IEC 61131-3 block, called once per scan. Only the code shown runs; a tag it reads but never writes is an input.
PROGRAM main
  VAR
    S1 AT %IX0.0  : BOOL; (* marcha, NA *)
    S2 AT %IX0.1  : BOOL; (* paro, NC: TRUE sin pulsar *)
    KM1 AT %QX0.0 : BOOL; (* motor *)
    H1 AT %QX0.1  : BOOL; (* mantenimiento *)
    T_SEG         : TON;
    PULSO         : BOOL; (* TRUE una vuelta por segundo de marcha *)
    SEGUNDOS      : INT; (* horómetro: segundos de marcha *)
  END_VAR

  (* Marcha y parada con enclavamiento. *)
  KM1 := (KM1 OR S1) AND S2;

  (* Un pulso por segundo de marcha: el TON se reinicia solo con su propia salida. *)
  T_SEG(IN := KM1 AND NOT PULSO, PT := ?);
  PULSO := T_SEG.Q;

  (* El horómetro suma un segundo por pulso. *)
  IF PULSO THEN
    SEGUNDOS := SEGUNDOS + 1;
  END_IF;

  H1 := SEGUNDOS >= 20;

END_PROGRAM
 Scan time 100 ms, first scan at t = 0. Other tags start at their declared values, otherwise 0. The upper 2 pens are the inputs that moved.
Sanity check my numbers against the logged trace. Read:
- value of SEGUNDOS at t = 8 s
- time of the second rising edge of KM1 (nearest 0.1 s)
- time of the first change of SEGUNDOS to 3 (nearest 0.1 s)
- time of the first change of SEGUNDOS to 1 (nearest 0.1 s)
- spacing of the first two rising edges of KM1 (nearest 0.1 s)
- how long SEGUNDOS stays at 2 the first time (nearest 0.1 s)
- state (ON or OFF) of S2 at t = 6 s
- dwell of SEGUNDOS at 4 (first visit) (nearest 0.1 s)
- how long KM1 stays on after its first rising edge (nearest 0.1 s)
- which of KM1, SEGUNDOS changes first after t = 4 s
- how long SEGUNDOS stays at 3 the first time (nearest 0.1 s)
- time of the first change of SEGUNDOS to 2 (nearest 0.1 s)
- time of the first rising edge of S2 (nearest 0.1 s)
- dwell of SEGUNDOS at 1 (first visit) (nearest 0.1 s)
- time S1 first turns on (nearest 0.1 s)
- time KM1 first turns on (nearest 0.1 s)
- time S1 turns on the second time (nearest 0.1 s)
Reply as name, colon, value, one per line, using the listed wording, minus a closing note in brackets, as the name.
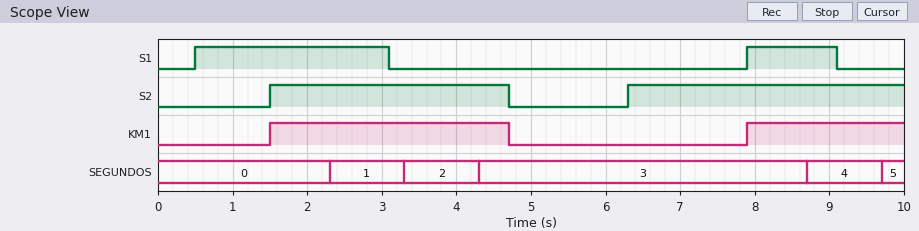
value of SEGUNDOS at t = 8 s: 3
time of the second rising edge of KM1: 7.9 s
time of the first change of SEGUNDOS to 3: 4.3 s
time of the first change of SEGUNDOS to 1: 2.3 s
spacing of the first two rising edges of KM1: 6.4 s
how long SEGUNDOS stays at 2 the first time: 1.0 s
state (ON or OFF) of S2 at t = 6 s: OFF
dwell of SEGUNDOS at 4 (first visit): 1.0 s
how long KM1 stays on after its first rising edge: 3.2 s
which of KM1, SEGUNDOS changes first after t = 4 s: SEGUNDOS
how long SEGUNDOS stays at 3 the first time: 4.4 s
time of the first change of SEGUNDOS to 2: 3.3 s
time of the first rising edge of S2: 1.5 s
dwell of SEGUNDOS at 1 (first visit): 1.0 s
time S1 first turns on: 0.5 s
time KM1 first turns on: 1.5 s
time S1 turns on the second time: 7.9 s
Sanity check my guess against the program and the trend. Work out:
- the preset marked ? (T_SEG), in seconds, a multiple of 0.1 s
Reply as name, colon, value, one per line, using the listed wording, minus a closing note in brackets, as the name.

the preset marked ? (T_SEG), in seconds, a multiple of 0.1 s: 0.8 s
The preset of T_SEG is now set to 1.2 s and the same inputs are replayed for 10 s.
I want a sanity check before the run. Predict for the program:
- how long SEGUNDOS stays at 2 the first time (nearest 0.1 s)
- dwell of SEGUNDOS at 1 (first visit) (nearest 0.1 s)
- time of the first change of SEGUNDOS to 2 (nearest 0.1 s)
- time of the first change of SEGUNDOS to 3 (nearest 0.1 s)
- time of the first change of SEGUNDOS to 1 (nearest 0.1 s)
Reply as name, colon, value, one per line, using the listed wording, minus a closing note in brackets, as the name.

how long SEGUNDOS stays at 2 the first time: 5.0 s
dwell of SEGUNDOS at 1 (first visit): 1.4 s
time of the first change of SEGUNDOS to 2: 4.1 s
time of the first change of SEGUNDOS to 3: 9.1 s
time of the first change of SEGUNDOS to 1: 2.7 s
